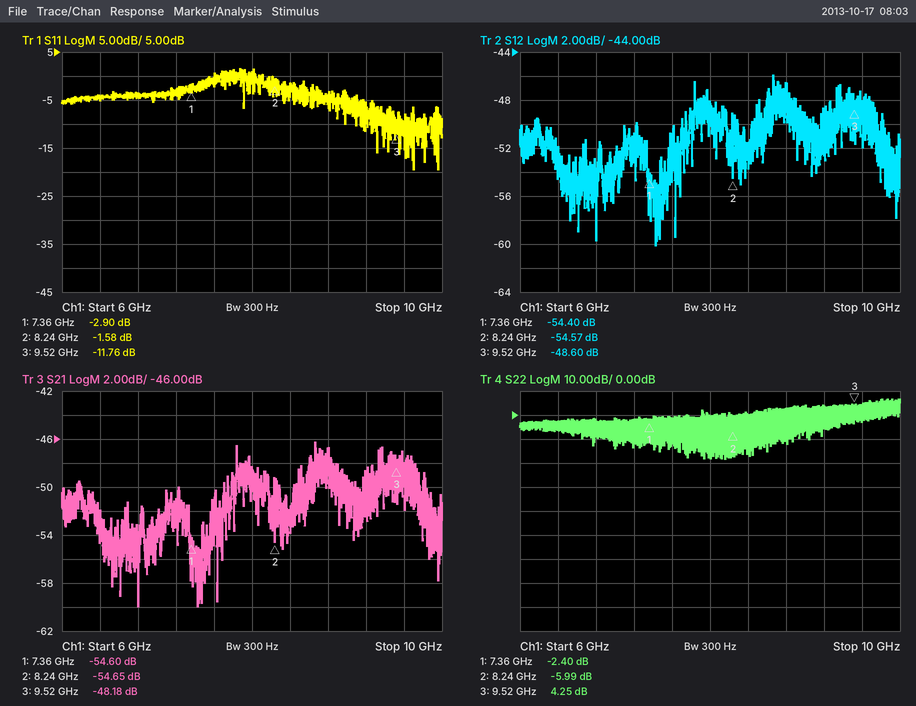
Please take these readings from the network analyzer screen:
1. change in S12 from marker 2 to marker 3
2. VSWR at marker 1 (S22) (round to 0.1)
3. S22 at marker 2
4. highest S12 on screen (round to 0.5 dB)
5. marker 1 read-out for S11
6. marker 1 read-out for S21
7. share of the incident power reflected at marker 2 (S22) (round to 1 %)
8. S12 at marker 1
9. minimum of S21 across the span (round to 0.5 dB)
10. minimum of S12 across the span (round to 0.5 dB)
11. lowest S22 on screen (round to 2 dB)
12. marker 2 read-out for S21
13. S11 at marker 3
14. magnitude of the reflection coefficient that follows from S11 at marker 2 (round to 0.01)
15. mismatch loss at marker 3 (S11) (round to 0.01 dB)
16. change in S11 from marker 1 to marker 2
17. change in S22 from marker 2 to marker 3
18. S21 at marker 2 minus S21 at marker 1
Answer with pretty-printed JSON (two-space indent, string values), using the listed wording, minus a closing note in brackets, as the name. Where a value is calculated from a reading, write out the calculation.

{
  "change in S12 from marker 2 to marker 3": "-48.6 − (-54.57) = 5.97 dB",
  "VSWR at marker 1 (S22)": "(1 + 0.7586)/(1 − 0.7586) ≈ 7.3",
  "S22 at marker 2": "-5.99 dB",
  "highest S12 on screen": "-46.0 dB",
  "marker 1 read-out for S11": "-2.90 dB",
  "marker 1 read-out for S21": "-54.60 dB",
  "share of the incident power reflected at marker 2 (S22)": "10^(-5.99/10) ≈ 25 %",
  "S12 at marker 1": "-54.40 dB",
  "minimum of S21 across the span": "-60.0 dB",
  "minimum of S12 across the span": "-60.0 dB",
  "lowest S22 on screen": "-18 dB",
  "marker 2 read-out for S21": "-54.65 dB",
  "S11 at marker 3": "-11.76 dB",
  "magnitude of the reflection coefficient that follows from S11 at marker 2": "10^(-1.58/20) ≈ 0.83",
  "mismatch loss at marker 3 (S11)": "−10 log10(1 − 10^(-11.76/10)) ≈ 0.30 dB",
  "change in S11 from marker 1 to marker 2": "-1.58 − (-2.9) = 1.32 dB",
  "change in S22 from marker 2 to marker 3": "4.25 − (-5.99) = 10.24 dB",
  "S21 at marker 2 minus S21 at marker 1": "-54.65 − (-54.6) = -0.05 dB"
}
